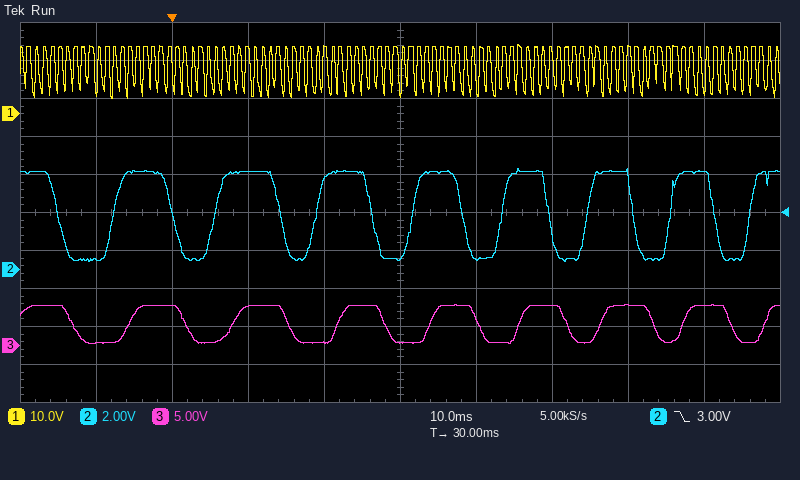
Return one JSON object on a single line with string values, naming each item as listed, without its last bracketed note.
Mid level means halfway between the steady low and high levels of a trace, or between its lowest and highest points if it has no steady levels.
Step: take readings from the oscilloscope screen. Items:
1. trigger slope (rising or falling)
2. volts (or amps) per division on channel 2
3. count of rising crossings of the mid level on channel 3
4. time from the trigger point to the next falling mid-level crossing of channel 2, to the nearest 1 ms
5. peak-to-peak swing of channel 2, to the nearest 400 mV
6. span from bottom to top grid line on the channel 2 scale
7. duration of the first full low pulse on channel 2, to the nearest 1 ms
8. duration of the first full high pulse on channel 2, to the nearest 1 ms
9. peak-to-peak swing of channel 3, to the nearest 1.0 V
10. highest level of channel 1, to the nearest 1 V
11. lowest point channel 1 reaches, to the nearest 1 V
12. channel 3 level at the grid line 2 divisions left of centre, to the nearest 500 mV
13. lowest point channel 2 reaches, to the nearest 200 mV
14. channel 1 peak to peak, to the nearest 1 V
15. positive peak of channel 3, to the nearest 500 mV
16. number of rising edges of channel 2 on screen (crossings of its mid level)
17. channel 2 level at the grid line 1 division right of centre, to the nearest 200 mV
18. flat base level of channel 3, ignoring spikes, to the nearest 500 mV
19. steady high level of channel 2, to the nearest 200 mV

{"trigger slope": "falling", "volts (or amps) per division on channel 2": "2 V", "count of rising crossings of the mid level on channel 3": "8", "time from the trigger point to the next falling mid-level crossing of channel 2, to the nearest 1 ms": "14 ms", "peak-to-peak swing of channel 2, to the nearest 400 mV": "4.8 V", "span from bottom to top grid line on the channel 2 scale": "20 V", "duration of the first full low pulse on channel 2, to the nearest 1 ms": "7 ms", "duration of the first full high pulse on channel 2, to the nearest 1 ms": "8 ms", "peak-to-peak swing of channel 3, to the nearest 1.0 V": "5.0 V", "highest level of channel 1, to the nearest 1 V": "18 V", "lowest point channel 1 reaches, to the nearest 1 V": "4 V", "channel 3 level at the grid line 2 divisions left of centre, to the nearest 500 mV": "5.0 V", "lowest point channel 2 reaches, to the nearest 200 mV": "400 mV", "channel 1 peak to peak, to the nearest 1 V": "14 V", "positive peak of channel 3, to the nearest 500 mV": "5.5 V", "number of rising edges of channel 2 on screen": "8", "channel 2 level at the grid line 1 division right of centre, to the nearest 200 mV": "600 mV", "flat base level of channel 3, ignoring spikes, to the nearest 500 mV": "500 mV", "steady high level of channel 2, to the nearest 200 mV": "5.2 V"}
